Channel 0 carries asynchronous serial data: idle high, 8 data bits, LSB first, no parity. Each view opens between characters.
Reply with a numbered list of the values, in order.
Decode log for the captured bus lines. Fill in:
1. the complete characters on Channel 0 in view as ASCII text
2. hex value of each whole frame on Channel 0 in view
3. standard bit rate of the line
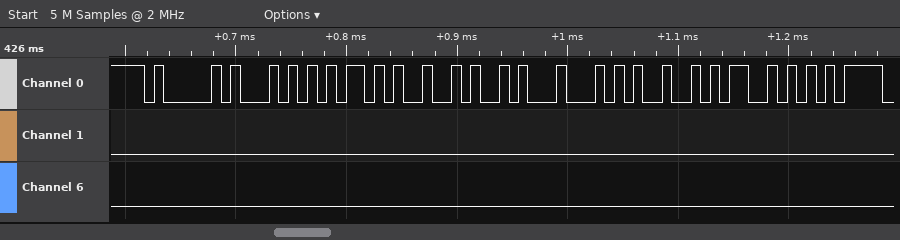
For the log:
1. "AT+JDIS"
2. 41, 54, 2B, 4A, 44, 49, 53
3. 115200 baud
